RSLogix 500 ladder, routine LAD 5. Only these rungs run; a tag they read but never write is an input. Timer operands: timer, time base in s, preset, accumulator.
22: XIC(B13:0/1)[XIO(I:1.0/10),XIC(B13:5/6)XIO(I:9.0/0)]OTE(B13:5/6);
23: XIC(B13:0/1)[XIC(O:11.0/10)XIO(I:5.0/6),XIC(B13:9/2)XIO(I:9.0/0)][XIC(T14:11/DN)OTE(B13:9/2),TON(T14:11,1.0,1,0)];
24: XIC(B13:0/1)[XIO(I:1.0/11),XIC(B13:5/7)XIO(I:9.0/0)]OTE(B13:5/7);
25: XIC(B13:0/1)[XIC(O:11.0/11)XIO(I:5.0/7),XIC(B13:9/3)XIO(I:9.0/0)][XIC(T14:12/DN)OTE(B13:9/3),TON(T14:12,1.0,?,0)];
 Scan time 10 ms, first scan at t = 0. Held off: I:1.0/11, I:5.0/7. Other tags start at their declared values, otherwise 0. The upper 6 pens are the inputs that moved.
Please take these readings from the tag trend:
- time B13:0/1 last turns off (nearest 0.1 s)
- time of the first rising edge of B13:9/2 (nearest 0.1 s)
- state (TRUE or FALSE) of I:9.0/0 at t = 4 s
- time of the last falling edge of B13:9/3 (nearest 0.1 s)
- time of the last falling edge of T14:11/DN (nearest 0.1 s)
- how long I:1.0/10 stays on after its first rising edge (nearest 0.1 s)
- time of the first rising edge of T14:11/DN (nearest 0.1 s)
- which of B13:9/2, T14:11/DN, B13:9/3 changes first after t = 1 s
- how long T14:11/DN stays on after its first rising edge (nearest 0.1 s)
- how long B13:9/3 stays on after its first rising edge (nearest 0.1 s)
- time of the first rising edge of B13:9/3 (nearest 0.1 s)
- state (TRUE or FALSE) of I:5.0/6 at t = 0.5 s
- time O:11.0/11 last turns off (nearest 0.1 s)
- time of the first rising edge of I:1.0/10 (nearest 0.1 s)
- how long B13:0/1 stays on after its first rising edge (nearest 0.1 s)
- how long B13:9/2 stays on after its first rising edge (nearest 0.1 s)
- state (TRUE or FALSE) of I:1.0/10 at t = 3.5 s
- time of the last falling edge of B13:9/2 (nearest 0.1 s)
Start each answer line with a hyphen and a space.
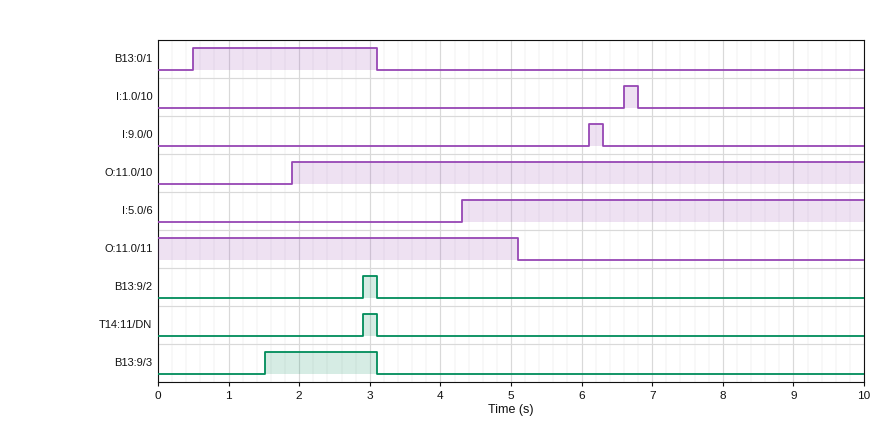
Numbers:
- 3.1 s
- 2.9 s
- FALSE
- 3.1 s
- 3.1 s
- 0.2 s
- 2.9 s
- B13:9/3
- 0.2 s
- 1.6 s
- 1.5 s
- FALSE
- 5.1 s
- 6.6 s
- 2.6 s
- 0.2 s
- FALSE
- 3.1 s
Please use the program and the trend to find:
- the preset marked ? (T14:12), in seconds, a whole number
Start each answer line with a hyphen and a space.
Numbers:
- 1 s
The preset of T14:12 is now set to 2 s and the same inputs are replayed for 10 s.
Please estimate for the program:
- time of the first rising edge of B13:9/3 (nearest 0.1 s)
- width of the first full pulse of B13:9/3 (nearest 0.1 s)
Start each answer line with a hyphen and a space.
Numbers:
- 2.5 s
- 0.6 s
